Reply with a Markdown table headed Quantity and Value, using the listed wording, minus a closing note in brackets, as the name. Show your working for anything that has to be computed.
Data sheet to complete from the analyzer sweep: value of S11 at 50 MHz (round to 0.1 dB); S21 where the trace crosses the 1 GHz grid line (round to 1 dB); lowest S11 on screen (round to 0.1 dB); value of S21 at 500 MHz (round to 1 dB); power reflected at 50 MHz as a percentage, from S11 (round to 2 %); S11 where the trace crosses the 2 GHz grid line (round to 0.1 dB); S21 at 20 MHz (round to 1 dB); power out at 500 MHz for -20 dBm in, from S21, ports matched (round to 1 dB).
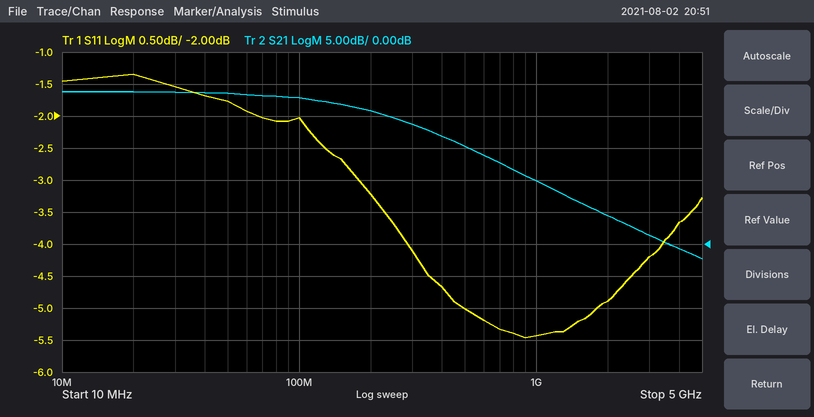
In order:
| Quantity | Value |
|---|---|
| value of S11 at 50 MHz | -1.8 dB |
| S21 where the trace crosses the 1 GHz grid line | 10 dB |
| lowest S11 on screen | -5.5 dB |
| value of S21 at 500 MHz | 15 dB |
| power reflected at 50 MHz as a percentage, from S11 | 10^(-1.8/10) ≈ 66 % |
| S11 where the trace crosses the 2 GHz grid line | -4.9 dB |
| S21 at 20 MHz | 24 dB |
| power out at 500 MHz for -20 dBm in, from S21, ports matched | -20 dBm + (15 dB) = -5 dBm |
